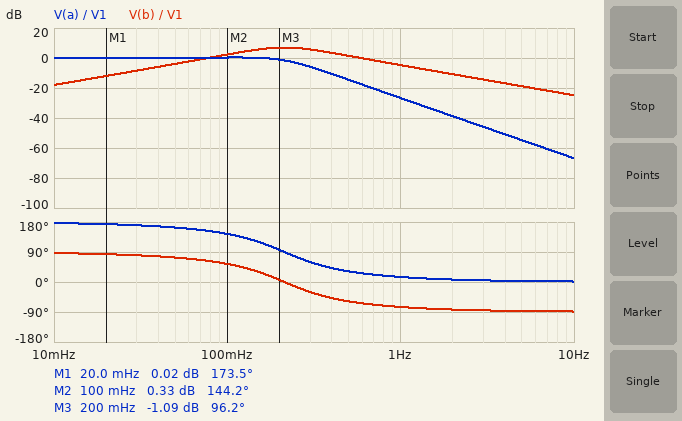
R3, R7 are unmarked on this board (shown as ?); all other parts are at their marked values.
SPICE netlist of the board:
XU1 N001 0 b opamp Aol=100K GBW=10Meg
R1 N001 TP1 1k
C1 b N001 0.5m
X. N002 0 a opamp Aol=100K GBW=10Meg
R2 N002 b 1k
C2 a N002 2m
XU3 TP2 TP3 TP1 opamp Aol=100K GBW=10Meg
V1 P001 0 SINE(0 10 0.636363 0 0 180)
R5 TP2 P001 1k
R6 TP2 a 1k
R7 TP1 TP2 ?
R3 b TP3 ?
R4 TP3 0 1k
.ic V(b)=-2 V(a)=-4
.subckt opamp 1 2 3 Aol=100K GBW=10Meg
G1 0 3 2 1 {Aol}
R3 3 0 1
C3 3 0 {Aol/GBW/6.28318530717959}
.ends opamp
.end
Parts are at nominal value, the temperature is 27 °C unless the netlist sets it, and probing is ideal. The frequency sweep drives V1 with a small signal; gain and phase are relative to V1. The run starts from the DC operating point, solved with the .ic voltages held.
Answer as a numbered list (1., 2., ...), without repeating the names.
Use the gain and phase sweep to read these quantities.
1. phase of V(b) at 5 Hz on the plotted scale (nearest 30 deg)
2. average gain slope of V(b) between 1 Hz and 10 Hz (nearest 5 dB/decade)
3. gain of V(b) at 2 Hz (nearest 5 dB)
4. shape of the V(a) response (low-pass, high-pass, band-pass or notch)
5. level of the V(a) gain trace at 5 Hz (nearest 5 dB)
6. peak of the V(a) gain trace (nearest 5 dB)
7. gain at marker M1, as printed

1. -90 deg
2. -20 dB/decade
3. -10 dB
4. low-pass
5. -55 dB
6. 0 dB
7. 0.02 dB
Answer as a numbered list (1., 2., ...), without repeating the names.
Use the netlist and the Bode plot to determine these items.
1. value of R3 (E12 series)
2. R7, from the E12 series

1. 4.7 kΩ
2. 1.8 kΩ
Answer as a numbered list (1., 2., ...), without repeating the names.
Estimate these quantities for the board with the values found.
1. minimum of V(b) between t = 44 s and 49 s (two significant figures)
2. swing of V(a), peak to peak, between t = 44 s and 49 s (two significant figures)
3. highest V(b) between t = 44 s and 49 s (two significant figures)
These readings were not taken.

1. -9.2 V
2. 2.3 V
3. 9.2 V
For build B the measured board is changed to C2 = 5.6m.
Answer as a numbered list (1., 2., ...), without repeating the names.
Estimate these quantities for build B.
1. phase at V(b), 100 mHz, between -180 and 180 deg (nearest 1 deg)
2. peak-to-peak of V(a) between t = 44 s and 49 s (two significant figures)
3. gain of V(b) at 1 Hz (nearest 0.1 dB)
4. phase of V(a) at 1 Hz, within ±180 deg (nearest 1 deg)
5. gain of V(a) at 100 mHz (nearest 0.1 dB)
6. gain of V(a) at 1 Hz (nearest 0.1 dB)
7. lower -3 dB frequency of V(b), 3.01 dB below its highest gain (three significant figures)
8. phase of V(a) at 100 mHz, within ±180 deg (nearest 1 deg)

1. 14 deg
2. 770 mV
3. -5.0 dB
4. 15 deg
5. -4.2 dB
6. -35.9 dB
7. 52.6 mHz
8. 104 deg
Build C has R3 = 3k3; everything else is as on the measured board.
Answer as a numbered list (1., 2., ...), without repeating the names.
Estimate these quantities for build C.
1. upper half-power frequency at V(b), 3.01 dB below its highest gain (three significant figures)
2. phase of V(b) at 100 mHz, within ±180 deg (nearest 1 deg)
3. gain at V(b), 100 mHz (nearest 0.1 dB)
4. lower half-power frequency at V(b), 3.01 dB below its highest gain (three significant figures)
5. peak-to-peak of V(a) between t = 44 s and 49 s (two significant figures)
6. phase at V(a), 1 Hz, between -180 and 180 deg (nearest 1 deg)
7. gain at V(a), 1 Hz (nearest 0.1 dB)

1. 443 mHz
2. 46 deg
3. 1.3 dB
4. 103 mHz
5. 2.2 V
6. 20 deg
7. -26.9 dB
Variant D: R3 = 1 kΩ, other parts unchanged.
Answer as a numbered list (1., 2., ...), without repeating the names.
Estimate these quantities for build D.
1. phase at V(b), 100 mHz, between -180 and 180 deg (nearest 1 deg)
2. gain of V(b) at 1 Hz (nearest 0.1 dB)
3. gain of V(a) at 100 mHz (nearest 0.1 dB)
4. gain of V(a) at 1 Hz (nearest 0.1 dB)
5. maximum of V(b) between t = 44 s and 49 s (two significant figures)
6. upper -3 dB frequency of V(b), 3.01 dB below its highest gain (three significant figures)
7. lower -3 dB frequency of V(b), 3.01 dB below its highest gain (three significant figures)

1. 26 deg
2. -6.4 dB
3. -5.0 dB
4. -28.4 dB
5. 6.2 V
6. 790 mHz
7. 57.7 mHz
